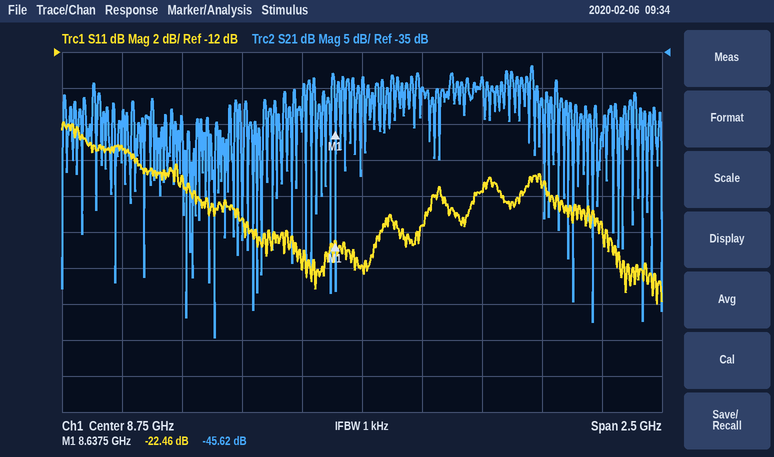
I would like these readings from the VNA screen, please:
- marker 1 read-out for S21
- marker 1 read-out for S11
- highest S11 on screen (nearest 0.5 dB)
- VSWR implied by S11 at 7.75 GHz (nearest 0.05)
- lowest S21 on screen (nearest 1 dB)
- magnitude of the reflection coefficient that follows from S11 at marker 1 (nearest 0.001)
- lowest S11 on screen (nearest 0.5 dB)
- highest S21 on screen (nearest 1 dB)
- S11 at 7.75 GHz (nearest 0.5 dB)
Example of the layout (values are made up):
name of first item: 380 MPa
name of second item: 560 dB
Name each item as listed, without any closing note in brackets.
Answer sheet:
marker 1 read-out for S21: -45.62 dB
marker 1 read-out for S11: -22.46 dB
highest S11 on screen: -16.0 dB
VSWR implied by S11 at 7.75 GHz: 1.30
lowest S21 on screen: -75 dB
magnitude of the reflection coefficient that follows from S11 at marker 1: 0.075
lowest S11 on screen: -26.0 dB
highest S21 on screen: -37 dB
S11 at 7.75 GHz: -17.5 dB
